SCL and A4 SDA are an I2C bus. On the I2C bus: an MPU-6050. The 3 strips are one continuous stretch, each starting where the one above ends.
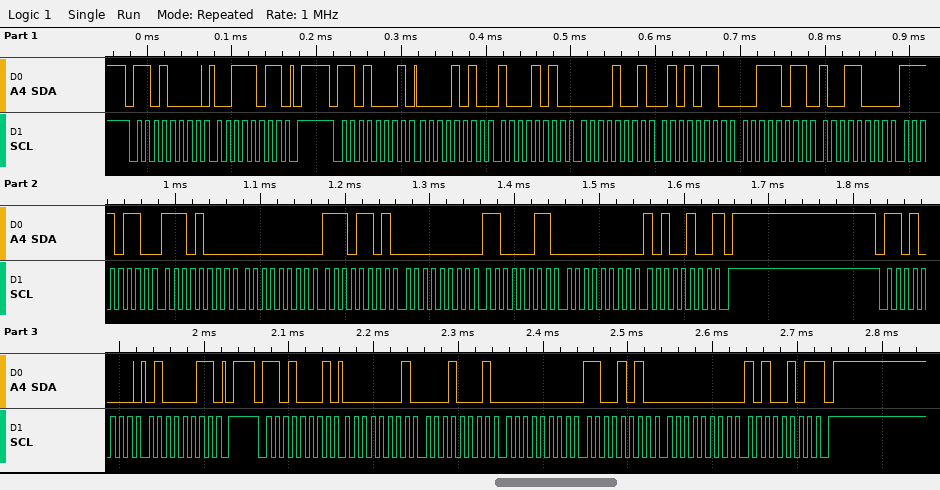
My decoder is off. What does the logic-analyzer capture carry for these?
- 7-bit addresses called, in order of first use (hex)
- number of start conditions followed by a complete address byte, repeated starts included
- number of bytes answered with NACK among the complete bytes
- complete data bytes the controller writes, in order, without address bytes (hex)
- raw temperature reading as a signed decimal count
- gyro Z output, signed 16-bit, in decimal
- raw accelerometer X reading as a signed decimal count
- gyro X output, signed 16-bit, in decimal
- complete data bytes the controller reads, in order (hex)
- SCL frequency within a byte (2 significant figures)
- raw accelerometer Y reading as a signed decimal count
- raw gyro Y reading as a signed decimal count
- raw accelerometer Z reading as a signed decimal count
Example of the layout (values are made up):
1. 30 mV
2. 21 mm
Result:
1. 0x68
2. 4
3. 2
4. 3B 43
5. -2328
6. 164
7. 2698
8. 237
9. 0A 8A 09 56 3B 98 F6 E8 00 ED 00 C3 00 A4 01 11 00 CA 00 A5
10. 100 kHz
11. 2390
12. 195
13. 15256
